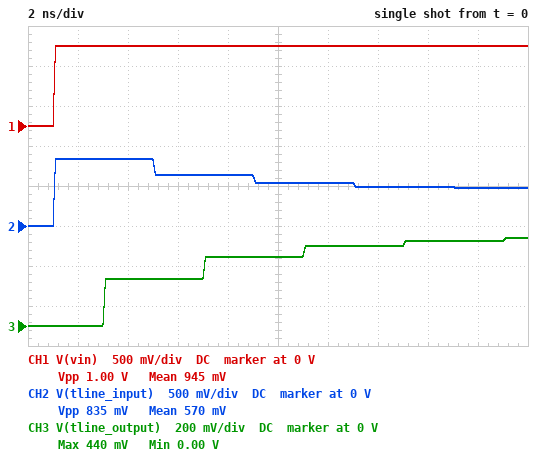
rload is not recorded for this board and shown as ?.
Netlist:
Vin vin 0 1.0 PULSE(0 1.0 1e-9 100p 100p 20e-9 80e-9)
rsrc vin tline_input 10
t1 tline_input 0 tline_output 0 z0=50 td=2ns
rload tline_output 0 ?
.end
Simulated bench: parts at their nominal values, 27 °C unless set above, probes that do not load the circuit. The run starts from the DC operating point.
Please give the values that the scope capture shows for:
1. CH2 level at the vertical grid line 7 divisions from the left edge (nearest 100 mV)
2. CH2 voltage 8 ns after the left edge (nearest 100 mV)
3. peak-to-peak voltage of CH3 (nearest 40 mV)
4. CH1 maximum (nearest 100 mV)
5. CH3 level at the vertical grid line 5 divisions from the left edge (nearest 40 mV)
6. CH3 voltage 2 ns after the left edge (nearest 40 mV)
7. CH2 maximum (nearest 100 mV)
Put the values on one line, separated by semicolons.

500 mV; 600 mV; 440 mV; 1.0 V; 360 mV; 0 V; 800 mV
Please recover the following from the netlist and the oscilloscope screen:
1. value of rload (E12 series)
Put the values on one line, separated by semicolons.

8.2 Ω
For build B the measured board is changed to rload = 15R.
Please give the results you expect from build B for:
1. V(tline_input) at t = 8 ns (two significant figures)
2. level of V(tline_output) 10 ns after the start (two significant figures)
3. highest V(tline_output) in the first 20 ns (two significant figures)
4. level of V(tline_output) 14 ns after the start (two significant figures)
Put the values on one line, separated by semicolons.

680 mV; 520 mV; 600 mV; 570 mV
